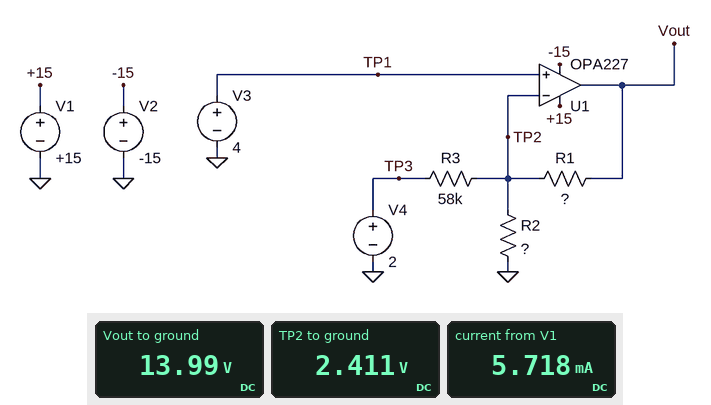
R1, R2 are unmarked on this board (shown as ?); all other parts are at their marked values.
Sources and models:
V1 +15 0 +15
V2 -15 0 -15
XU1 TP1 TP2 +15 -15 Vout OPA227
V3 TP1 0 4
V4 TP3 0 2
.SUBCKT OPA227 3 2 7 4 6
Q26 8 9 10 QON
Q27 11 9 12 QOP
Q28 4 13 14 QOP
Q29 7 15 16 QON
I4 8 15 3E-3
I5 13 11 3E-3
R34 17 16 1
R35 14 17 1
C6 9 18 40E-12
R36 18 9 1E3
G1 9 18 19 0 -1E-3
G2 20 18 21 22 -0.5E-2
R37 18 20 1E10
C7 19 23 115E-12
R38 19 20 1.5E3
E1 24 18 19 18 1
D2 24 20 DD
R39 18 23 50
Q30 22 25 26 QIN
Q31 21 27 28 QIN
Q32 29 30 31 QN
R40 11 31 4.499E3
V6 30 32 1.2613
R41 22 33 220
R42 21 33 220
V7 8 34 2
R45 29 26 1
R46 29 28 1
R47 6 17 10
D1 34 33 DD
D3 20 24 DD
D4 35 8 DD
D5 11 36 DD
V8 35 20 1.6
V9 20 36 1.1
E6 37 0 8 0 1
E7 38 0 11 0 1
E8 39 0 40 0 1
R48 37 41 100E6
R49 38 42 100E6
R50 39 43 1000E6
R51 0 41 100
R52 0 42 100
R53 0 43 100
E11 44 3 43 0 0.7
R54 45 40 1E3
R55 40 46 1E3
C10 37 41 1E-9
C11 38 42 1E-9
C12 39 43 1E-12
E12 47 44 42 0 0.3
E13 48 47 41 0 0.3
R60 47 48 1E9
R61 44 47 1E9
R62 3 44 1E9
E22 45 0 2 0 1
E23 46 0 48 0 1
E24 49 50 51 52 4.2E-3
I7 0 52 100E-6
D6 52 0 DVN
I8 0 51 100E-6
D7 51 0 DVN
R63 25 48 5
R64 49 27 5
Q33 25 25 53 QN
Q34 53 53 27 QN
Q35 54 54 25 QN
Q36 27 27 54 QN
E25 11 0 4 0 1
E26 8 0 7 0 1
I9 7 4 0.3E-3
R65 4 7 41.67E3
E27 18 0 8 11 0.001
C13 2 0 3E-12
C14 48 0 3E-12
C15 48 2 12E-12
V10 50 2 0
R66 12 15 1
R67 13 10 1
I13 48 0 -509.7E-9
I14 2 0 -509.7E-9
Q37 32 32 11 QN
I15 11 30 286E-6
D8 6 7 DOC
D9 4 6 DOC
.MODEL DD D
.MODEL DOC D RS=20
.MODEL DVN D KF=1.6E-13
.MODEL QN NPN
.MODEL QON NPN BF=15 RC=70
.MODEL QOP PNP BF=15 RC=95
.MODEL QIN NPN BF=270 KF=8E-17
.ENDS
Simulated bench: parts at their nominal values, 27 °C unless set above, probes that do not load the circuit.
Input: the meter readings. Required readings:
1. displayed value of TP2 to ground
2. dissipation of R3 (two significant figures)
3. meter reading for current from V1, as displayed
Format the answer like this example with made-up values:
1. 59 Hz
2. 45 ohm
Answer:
1. 2.411 V
2. 2.9 µW
3. 5.718 mA
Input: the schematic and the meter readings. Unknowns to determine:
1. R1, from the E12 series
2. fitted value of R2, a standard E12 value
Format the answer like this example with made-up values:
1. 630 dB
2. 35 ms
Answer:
1. 3.3 kΩ
2. 470 Ω
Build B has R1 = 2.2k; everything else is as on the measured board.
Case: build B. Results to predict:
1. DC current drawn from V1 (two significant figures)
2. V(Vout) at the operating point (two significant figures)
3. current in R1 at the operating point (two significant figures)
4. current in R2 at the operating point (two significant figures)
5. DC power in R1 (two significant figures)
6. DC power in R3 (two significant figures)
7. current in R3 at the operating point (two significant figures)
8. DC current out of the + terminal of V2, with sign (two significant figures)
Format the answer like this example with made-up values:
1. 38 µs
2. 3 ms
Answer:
1. 6.9 mA
2. 14 V
3. 5.2 mA
4. 5.4 mA
5. 59 mW
6. 4.9 µW
7. 9.2 µA
8. -2.1 mA
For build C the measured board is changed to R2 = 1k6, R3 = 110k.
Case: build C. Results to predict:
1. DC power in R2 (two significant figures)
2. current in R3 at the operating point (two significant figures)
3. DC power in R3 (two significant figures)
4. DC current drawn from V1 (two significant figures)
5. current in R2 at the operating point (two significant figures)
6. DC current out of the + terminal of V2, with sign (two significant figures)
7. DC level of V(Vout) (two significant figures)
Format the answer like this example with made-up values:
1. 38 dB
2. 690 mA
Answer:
1. 10 mW
2. 18 µA
3. 36 µW
4. 5.1 mA
5. 2.5 mA
6. -2.7 mA
7. 12 V
